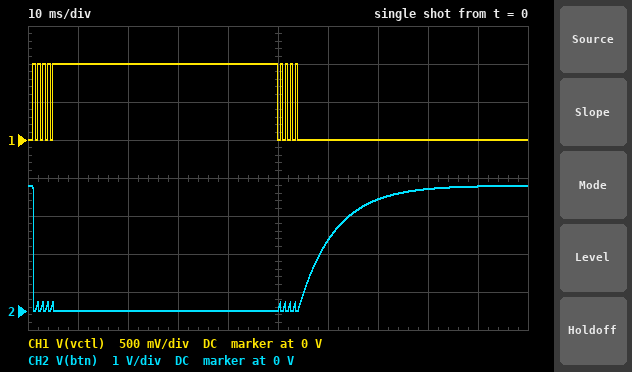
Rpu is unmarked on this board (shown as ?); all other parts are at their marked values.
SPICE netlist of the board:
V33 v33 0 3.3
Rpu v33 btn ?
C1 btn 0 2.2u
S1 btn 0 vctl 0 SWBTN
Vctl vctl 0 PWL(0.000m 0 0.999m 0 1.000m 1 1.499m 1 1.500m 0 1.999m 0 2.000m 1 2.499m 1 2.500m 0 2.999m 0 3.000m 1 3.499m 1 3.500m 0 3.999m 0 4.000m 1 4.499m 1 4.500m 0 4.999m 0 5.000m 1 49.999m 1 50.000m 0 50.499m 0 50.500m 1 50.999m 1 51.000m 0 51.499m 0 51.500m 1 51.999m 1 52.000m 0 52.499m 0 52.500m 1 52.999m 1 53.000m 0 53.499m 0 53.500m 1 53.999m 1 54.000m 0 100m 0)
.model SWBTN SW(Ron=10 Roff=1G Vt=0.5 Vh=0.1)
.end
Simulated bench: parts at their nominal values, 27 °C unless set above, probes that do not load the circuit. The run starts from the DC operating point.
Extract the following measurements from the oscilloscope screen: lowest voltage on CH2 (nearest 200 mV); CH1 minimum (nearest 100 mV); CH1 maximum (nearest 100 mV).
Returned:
0 V
0 V
1.0 V
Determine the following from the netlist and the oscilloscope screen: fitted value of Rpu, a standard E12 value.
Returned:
3.3 kΩ
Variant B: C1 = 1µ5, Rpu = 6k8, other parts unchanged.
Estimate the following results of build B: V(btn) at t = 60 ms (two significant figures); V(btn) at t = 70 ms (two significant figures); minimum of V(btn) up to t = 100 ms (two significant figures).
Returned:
1.5 V
2.6 V
4.8 mV
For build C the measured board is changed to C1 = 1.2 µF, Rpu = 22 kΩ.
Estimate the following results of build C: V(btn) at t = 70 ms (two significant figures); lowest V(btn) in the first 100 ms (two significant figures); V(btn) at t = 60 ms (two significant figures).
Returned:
1.5 V
1.5 mV
670 mV
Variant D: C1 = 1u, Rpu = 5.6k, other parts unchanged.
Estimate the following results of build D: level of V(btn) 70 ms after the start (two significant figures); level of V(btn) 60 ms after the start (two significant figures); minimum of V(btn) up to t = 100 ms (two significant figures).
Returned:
3.1 V
2.2 V
5.9 mV
